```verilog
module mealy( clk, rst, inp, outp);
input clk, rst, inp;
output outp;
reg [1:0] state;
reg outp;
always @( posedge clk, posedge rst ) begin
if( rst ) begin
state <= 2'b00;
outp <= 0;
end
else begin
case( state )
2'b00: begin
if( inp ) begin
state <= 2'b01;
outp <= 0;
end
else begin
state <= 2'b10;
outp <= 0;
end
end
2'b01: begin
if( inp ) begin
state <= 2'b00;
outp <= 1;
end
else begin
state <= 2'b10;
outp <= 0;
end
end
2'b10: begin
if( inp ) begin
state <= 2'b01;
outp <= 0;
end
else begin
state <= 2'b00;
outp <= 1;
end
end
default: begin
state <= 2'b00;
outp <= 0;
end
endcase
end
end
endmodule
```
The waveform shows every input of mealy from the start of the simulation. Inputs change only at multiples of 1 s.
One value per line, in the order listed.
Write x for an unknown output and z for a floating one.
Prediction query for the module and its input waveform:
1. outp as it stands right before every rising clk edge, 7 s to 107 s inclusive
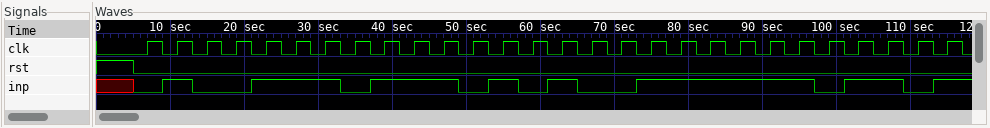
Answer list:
0 0 0 0 1 0 1 0 0 0 1 0 0 0 0 0 0 1 0 1 0 1 0 1 0 0
